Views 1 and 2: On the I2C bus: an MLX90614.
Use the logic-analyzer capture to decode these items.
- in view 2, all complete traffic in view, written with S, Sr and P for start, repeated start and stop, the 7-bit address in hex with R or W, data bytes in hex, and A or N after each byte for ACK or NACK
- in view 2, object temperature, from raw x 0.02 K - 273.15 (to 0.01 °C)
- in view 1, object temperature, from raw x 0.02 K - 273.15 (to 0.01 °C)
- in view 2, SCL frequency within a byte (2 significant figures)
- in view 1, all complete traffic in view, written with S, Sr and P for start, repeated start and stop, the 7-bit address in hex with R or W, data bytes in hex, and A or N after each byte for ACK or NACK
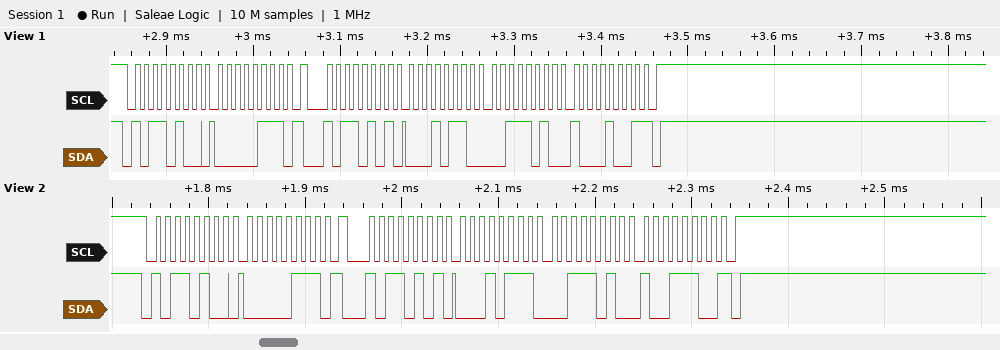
S 5AW A 07 A Sr 5AR A 17 A 3A A 9C N P
24.27 °C
24.25 °C
100 kHz
S 5AW A 07 A Sr 5AR A 16 A 3A A 89 N P
